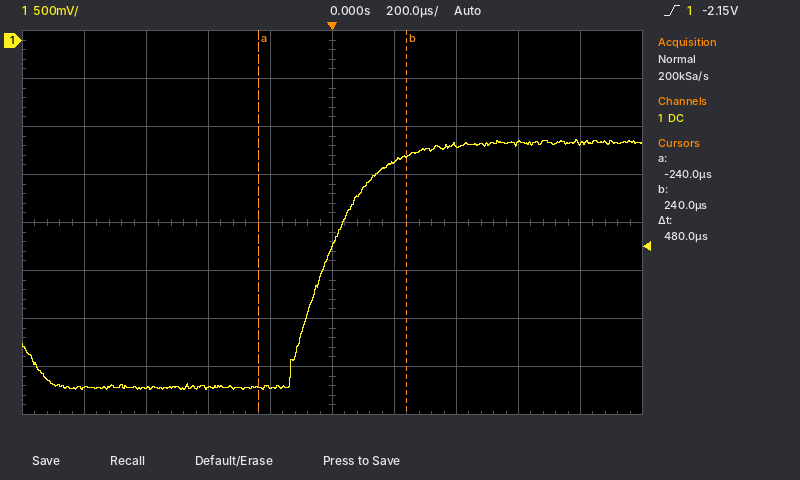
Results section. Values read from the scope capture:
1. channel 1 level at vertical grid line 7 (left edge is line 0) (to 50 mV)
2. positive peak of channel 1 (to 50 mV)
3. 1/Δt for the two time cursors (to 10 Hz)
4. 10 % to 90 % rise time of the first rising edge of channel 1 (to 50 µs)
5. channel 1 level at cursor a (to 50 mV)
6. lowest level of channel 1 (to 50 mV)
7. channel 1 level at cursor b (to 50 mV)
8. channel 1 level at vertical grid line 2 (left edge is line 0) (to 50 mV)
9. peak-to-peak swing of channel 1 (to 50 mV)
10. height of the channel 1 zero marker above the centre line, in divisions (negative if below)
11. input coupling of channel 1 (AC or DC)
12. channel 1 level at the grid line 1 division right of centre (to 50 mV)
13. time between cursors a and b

-1.10 V
-1.05 V
2.08 kHz
300 µs
-3.60 V
-3.65 V
-1.20 V
-3.60 V
2.60 V
+3.8 div
DC
-1.25 V
480 µs
